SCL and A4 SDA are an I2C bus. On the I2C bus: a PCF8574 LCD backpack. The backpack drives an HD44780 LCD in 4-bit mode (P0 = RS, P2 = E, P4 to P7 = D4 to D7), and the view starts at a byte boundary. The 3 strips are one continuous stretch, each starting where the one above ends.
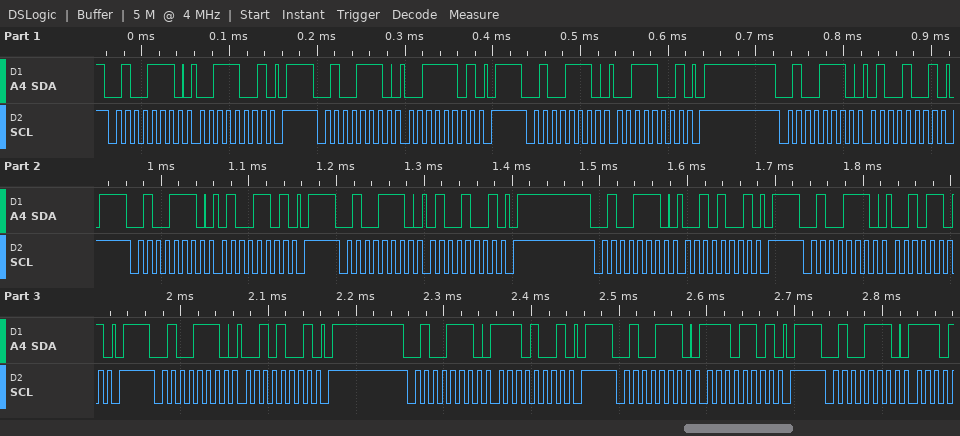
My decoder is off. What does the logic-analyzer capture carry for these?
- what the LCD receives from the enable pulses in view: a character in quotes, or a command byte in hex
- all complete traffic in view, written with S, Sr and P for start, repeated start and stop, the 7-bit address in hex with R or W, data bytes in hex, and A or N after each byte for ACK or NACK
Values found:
'4'
S 27W A 39 A P S 27W A 3D A P S 27W A 39 A P S 27W A 49 A P S 27W A 4D A P S 27W A 49 A P S 27W A 29 A P S 27W A 2D A P S 27W A 29 A P S 27W A E9 A P S 27W A ED A P S 27W A
